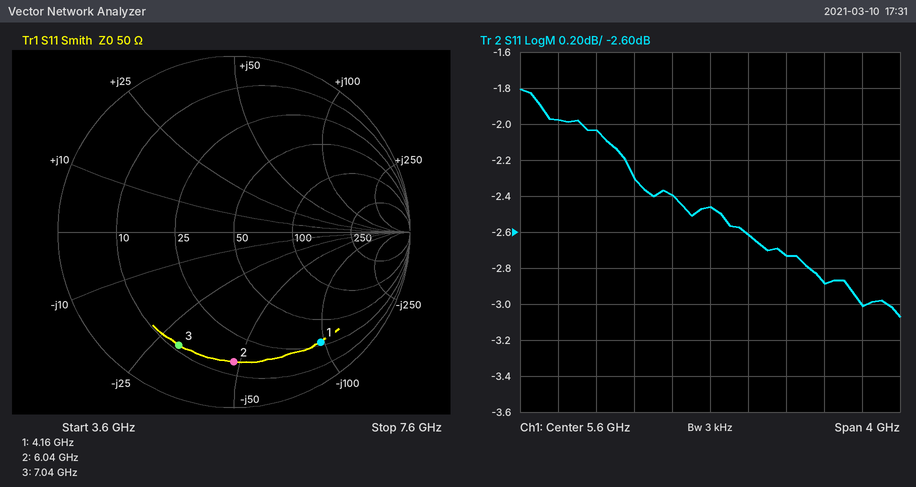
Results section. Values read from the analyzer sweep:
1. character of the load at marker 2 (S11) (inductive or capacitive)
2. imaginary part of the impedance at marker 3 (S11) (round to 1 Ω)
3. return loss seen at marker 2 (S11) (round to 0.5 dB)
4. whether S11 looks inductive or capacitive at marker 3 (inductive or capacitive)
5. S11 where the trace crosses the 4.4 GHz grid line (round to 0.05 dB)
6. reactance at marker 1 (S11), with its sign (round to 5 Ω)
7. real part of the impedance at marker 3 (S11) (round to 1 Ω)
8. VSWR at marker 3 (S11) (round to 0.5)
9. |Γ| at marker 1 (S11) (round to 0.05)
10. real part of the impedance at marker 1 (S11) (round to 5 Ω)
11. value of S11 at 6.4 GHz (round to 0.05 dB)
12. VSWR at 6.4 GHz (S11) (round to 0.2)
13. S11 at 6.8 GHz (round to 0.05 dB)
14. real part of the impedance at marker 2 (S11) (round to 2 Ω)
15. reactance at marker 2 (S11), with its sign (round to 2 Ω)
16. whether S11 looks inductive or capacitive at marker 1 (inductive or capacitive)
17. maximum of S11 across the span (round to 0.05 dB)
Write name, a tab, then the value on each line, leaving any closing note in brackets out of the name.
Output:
character of the load at marker 2 (S11)	capacitive
imaginary part of the impedance at marker 3 (S11)	-30 Ω
return loss seen at marker 2 (S11)	2.5 dB
whether S11 looks inductive or capacitive at marker 3	capacitive
S11 where the trace crosses the 4.4 GHz grid line	-2.05 dB
reactance at marker 1 (S11), with its sign	-95 Ω
real part of the impedance at marker 3 (S11)	11 Ω
VSWR at marker 3 (S11)	6.0
|Γ| at marker 1 (S11)	0.80
real part of the impedance at marker 1 (S11)	30 Ω
value of S11 at 6.4 GHz	-2.75 dB
VSWR at 6.4 GHz (S11)	6.4
S11 at 6.8 GHz	-2.90 dB
real part of the impedance at marker 2 (S11)	14 Ω
reactance at marker 2 (S11), with its sign	-48 Ω
whether S11 looks inductive or capacitive at marker 1	capacitive
maximum of S11 across the span	-1.80 dB
